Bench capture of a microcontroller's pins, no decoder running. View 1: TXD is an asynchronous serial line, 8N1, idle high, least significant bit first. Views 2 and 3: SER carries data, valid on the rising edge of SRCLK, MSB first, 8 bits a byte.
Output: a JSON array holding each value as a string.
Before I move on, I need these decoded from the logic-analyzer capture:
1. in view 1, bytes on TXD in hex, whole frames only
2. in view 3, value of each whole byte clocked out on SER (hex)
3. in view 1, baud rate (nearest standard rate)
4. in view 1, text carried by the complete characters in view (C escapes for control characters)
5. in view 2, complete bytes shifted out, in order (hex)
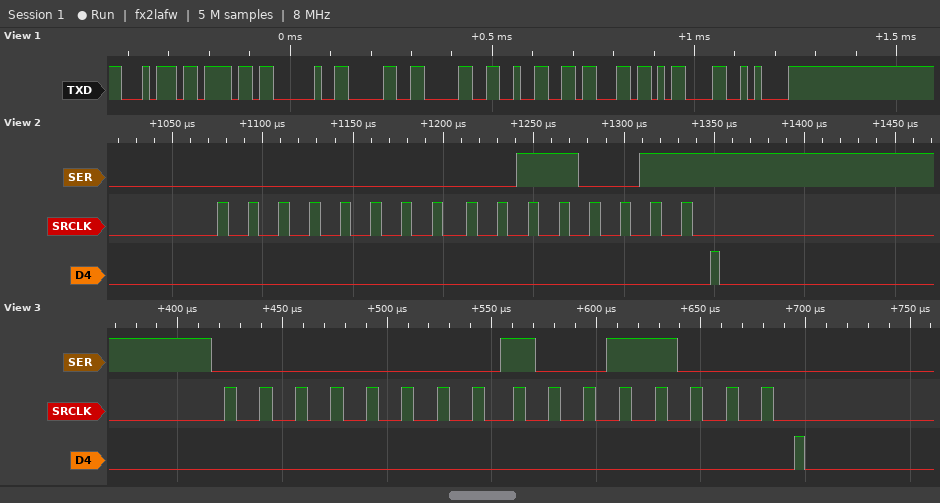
["74 6F 20 30 30 32 63 0D 0A", "00 98", "57600 baud", "\"to 002c\\r\\n\"", "00 33"]
